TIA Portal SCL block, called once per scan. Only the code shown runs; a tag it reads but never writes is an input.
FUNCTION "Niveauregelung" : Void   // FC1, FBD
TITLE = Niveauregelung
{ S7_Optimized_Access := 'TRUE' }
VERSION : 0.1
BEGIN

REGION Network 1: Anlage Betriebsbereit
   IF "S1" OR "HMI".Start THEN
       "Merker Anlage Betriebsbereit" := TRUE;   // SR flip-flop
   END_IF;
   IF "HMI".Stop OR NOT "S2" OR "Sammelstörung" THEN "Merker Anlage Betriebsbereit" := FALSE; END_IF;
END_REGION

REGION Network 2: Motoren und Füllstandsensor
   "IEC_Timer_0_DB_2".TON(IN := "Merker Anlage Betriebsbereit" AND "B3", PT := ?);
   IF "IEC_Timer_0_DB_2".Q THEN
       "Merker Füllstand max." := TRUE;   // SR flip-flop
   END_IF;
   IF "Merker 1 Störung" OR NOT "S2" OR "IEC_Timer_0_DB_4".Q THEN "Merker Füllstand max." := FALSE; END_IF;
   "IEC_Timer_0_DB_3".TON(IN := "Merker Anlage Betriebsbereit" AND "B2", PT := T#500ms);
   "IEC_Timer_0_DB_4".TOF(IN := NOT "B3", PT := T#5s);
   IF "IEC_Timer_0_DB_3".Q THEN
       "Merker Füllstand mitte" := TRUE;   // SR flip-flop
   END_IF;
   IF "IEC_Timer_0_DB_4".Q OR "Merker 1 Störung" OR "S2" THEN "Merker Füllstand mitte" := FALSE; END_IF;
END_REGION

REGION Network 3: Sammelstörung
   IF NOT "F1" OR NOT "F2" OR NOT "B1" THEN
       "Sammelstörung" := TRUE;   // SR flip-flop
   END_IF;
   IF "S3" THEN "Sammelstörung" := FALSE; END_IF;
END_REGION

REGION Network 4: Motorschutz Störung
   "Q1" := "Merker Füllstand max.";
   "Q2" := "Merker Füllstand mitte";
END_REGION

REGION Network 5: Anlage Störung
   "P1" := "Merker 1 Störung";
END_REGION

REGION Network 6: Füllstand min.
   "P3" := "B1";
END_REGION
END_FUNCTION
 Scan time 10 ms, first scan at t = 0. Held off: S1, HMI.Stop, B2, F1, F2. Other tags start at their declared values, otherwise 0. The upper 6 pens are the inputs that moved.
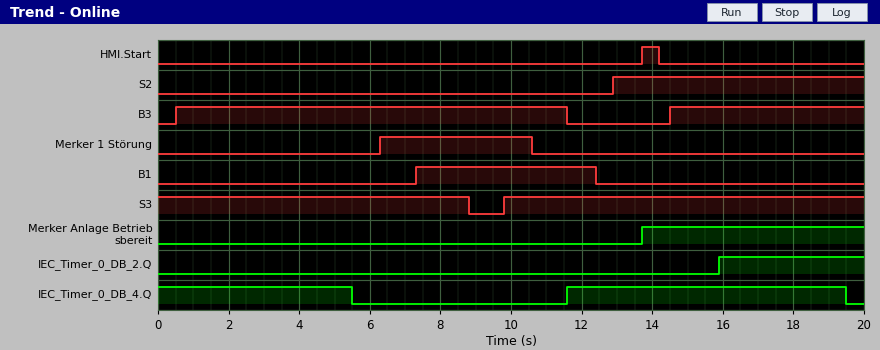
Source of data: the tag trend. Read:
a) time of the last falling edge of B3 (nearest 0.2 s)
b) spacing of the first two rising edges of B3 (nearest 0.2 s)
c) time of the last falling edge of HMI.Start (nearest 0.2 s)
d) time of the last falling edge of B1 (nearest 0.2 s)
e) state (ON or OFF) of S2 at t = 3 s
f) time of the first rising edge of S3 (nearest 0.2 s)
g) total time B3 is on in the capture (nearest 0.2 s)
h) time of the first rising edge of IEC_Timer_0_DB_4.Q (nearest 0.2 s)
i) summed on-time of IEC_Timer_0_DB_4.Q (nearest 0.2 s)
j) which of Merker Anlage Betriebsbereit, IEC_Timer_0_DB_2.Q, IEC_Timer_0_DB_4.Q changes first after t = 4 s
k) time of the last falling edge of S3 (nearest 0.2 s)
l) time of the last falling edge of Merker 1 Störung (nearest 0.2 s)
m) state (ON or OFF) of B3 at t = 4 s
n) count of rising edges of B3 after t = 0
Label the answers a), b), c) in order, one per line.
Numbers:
a) 11.6 s
b) 14.0 s
c) 14.2 s
d) 12.4 s
e) OFF
f) 9.8 s
g) 16.6 s
h) 11.6 s
i) 13.4 s
j) IEC_Timer_0_DB_4.Q
k) 8.8 s
l) 10.6 s
m) ON
n) 2
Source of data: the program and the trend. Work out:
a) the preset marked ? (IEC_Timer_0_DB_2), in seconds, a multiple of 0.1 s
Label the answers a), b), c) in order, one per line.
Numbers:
a) 1.4 s
